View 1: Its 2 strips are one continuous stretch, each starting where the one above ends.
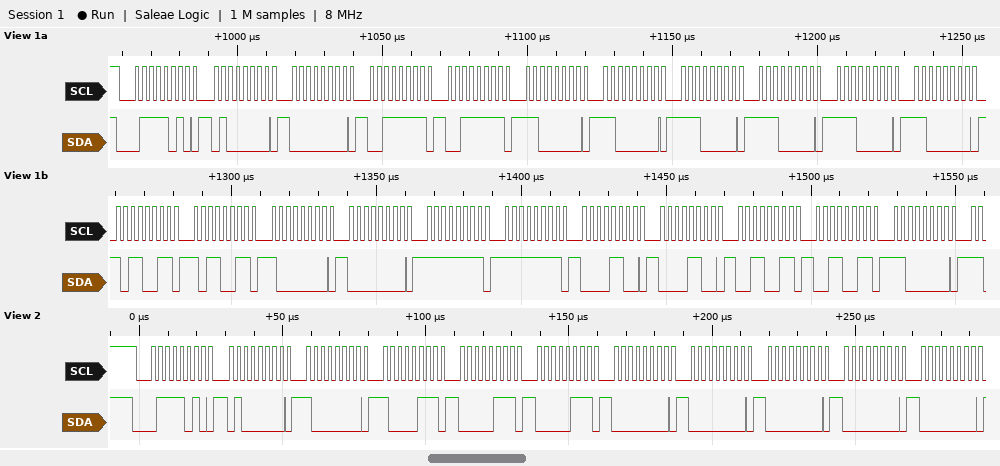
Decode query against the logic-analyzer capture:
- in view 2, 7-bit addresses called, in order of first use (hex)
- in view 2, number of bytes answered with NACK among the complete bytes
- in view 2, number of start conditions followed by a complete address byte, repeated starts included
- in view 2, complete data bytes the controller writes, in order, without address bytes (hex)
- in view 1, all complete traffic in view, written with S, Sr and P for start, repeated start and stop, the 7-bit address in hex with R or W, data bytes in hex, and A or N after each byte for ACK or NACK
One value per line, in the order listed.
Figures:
0x3D
0
1
40 80 87 07 07 00 00 00 00 00
S 3DW A 40 A 00 A 3F A 3F A C0 A C0 A E0 A E0 A E0 A C0 A B3 A B3 A 80 A 00 A FF A FF A 0C A 0C A 33 A 33 A C0 A
